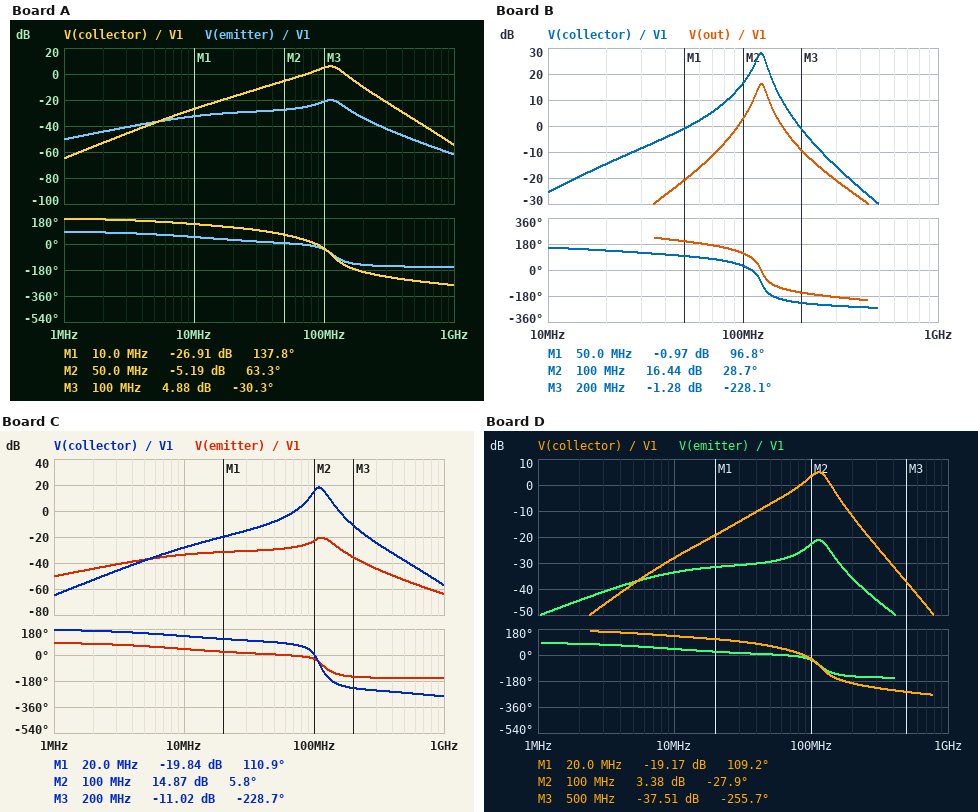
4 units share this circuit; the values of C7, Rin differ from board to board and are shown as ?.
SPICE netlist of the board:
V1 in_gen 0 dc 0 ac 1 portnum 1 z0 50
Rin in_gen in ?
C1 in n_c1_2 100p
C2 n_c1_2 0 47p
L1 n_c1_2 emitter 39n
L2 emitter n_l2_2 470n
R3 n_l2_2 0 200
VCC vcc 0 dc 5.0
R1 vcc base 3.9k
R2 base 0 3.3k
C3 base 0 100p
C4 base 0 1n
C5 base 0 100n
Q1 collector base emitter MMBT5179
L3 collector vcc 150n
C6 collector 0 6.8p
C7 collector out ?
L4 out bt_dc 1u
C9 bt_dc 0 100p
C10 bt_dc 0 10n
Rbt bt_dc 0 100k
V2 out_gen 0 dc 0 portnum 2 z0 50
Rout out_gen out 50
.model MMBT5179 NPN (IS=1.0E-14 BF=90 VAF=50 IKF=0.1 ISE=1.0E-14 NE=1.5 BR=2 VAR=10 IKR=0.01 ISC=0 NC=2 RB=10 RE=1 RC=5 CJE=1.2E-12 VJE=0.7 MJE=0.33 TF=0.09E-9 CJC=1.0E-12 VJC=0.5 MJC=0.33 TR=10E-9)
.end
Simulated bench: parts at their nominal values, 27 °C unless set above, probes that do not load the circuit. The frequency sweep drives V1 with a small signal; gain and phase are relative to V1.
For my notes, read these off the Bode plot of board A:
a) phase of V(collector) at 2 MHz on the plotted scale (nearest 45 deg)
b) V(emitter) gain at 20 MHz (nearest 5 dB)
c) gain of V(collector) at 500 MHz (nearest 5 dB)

180 deg
-30 dB
-35 dB
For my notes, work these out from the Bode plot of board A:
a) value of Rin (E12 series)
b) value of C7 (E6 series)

82 Ω
33 pF
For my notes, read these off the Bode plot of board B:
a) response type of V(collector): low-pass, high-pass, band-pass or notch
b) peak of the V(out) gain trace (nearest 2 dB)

band-pass
16 dB
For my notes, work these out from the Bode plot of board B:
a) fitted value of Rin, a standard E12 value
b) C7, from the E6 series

15 Ω
3.3 pF
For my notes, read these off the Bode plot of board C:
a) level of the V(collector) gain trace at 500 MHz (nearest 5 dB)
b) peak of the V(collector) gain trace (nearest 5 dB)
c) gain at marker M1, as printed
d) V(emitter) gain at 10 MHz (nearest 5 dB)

-40 dB
20 dB
-19.84 dB
-35 dB
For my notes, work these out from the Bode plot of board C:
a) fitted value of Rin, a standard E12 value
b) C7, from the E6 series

120 Ω
6.8 pF
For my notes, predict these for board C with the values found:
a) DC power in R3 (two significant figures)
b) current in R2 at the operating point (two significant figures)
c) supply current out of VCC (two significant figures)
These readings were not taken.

10 mW
650 µA
7.8 mA
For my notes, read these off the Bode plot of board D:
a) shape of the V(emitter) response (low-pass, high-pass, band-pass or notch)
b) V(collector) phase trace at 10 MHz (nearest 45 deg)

band-pass
135 deg
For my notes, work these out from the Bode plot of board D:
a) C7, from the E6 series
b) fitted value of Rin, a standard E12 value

33 pF
120 Ω
